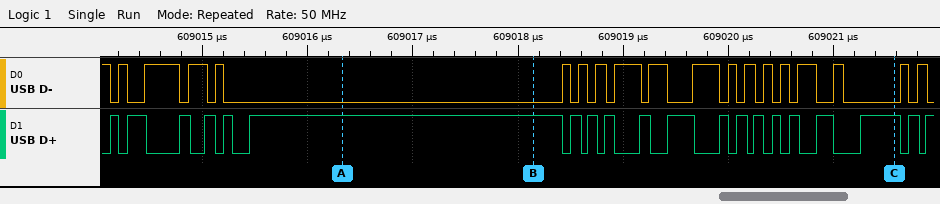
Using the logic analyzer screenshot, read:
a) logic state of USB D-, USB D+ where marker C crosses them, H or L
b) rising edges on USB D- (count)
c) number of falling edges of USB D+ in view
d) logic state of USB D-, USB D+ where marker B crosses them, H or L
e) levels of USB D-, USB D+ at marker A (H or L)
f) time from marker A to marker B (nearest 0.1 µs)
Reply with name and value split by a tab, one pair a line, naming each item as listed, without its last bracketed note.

logic state of USB D-, USB D+ where marker C crosses them, H or L	USB D-=L, USB D+=H
rising edges on USB D-	18
number of falling edges of USB D+ in view	19
logic state of USB D-, USB D+ where marker B crosses them, H or L	USB D-=L, USB D+=H
levels of USB D-, USB D+ at marker A	USB D-=L, USB D+=H
time from marker A to marker B	1.8 µs
